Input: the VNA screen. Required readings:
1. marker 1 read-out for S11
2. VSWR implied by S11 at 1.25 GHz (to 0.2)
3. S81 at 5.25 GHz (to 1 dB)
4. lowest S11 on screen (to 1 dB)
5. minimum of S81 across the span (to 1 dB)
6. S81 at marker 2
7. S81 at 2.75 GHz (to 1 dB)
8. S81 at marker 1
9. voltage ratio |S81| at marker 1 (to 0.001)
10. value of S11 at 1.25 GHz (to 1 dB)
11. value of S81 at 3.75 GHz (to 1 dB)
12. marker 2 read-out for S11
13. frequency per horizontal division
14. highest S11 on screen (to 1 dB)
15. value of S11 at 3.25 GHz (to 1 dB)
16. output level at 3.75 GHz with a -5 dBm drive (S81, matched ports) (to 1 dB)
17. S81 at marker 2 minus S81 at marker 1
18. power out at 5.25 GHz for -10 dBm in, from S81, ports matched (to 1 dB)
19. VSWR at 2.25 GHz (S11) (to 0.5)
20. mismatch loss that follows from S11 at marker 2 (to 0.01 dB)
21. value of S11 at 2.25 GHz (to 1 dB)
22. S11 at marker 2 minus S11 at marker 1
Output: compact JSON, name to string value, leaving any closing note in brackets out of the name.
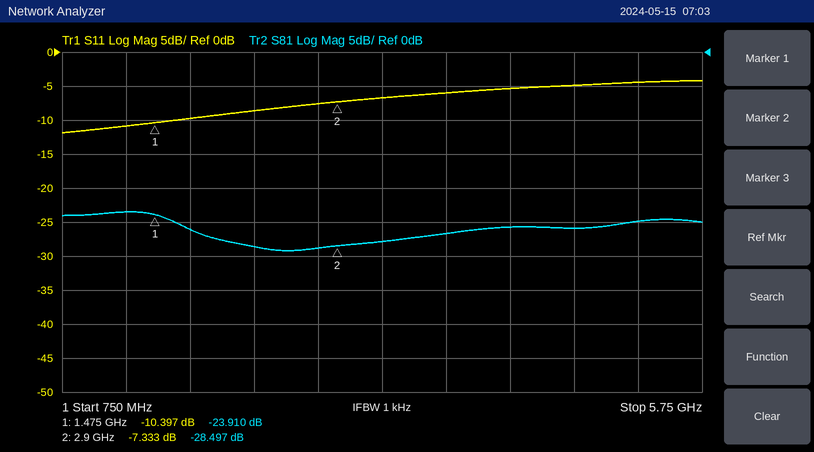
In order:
{"marker 1 read-out for S11": "-10.397 dB", "VSWR implied by S11 at 1.25 GHz": "1.8", "S81 at 5.25 GHz": "-25 dB", "lowest S11 on screen": "-12 dB", "minimum of S81 across the span": "-29 dB", "S81 at marker 2": "-28.497 dB", "S81 at 2.75 GHz": "-29 dB", "S81 at marker 1": "-23.910 dB", "voltage ratio |S81| at marker 1": "0.064", "value of S11 at 1.25 GHz": "-11 dB", "value of S81 at 3.75 GHz": "-27 dB", "marker 2 read-out for S11": "-7.333 dB", "frequency per horizontal division": "500 MHz", "highest S11 on screen": "-4 dB", "value of S11 at 3.25 GHz": "-7 dB", "output level at 3.75 GHz with a -5 dBm drive (S81, matched ports)": "-32 dBm", "S81 at marker 2 minus S81 at marker 1": "-4.587 dB", "power out at 5.25 GHz for -10 dBm in, from S81, ports matched": "-35 dBm", "VSWR at 2.25 GHz (S11)": "2.0", "mismatch loss that follows from S11 at marker 2": "0.89 dB", "value of S11 at 2.25 GHz": "-9 dB", "S11 at marker 2 minus S11 at marker 1": "3.064 dB"}
